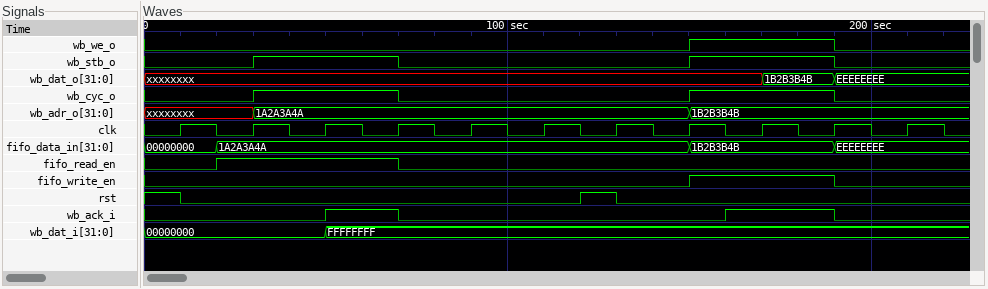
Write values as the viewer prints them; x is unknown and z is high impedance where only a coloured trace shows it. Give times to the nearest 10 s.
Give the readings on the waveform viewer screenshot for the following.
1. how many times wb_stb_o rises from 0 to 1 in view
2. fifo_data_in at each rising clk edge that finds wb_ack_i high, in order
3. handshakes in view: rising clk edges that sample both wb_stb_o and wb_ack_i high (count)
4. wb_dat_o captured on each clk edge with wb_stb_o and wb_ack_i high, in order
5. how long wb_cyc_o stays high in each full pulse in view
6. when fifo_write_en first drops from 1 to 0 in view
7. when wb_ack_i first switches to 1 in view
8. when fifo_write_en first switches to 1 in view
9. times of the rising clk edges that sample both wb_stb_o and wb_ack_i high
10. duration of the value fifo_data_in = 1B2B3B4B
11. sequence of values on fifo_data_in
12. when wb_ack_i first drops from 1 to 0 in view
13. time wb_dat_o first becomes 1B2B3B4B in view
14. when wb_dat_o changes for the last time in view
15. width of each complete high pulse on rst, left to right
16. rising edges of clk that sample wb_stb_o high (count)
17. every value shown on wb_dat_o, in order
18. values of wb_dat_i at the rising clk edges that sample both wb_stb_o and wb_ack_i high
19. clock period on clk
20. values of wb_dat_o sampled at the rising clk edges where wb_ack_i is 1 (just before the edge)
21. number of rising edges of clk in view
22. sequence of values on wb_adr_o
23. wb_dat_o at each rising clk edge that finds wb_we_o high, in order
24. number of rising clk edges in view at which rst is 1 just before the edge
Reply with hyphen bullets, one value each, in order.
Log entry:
- 2
- 1A2A3A4A, 1B2B3B4B, 1B2B3B4B
- 3
- xxxxxxxx, xxxxxxxx, 1B2B3B4B
- 40 s, 40 s
- 190 s
- 50 s
- 150 s
- 70 s, 170 s, 190 s
- 40 s
- 00000000, 1A2A3A4A, 1B2B3B4B, EEEEEEEE
- 70 s
- 170 s
- 190 s
- 10 s
- 4
- xxxxxxxx, 1B2B3B4B, EEEEEEEE
- FFFFFFFF, FFFFFFFF, FFFFFFFF
- 20 s
- xxxxxxxx, xxxxxxxx, 1B2B3B4B
- 11
- xxxxxxxx, 1A2A3A4A, 1B2B3B4B
- xxxxxxxx, 1B2B3B4B
- 2
